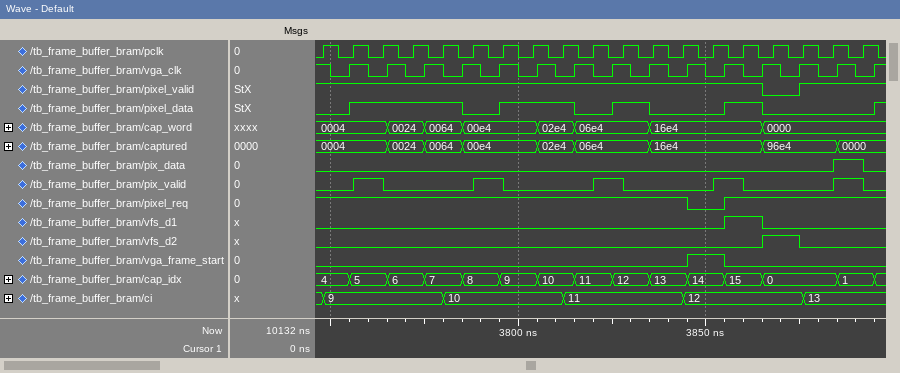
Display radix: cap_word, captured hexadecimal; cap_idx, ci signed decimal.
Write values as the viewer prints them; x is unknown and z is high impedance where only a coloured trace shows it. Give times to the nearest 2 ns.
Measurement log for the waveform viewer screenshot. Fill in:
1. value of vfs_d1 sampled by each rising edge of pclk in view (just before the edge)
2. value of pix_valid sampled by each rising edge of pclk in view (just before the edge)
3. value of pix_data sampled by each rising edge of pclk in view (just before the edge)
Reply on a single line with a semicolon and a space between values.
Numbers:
0 0 0 0 0 0 0 0 0 0 0 0 0 0 1 0 0 0 0; 0 0 1 0 0 0 1 0 0 0 1 0 0 0 1 0 0 0 1; 0 0 0 0 0 0 0 0 0 0 0 0 0 0 0 0 0 0 1
